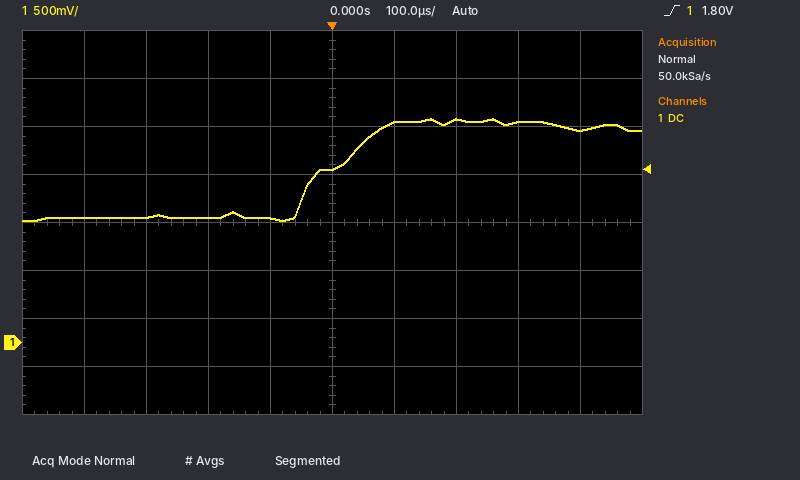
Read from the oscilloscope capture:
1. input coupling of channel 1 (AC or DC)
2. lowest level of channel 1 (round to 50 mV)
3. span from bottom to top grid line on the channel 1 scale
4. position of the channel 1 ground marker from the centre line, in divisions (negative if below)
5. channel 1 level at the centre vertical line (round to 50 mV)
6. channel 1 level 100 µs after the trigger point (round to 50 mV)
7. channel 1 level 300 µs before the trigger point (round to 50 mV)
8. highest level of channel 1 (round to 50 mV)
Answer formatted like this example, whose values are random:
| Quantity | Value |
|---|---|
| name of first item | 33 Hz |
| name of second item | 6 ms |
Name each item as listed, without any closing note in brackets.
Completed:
| Quantity | Value |
|---|---|
| input coupling of channel 1 | DC |
| lowest level of channel 1 | 1.25 V |
| span from bottom to top grid line on the channel 1 scale | 4 V |
| position of the channel 1 ground marker from the centre line, in divisions | -2.5 div |
| channel 1 level at the centre vertical line | 1.80 V |
| channel 1 level 100 µs after the trigger point | 2.30 V |
| channel 1 level 300 µs before the trigger point | 1.30 V |
| highest level of channel 1 | 2.35 V |
